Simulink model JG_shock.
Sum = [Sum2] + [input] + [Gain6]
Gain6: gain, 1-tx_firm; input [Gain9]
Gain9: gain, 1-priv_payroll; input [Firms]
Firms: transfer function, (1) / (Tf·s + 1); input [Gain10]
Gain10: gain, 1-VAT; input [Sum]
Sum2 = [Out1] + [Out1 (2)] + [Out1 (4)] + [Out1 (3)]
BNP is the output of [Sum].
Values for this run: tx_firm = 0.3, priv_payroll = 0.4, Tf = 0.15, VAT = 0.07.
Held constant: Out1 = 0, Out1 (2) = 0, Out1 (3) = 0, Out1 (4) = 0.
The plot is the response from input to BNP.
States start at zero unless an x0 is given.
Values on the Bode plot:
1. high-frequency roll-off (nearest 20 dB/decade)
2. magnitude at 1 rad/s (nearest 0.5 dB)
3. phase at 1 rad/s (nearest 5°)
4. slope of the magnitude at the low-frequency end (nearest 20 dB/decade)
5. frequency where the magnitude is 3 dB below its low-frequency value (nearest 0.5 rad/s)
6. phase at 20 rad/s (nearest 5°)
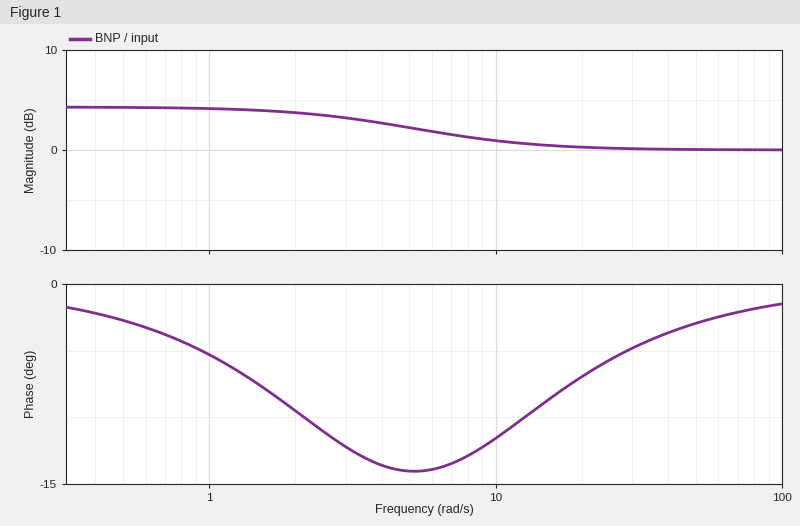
0 dB/decade
4.0 dB
-5°
0 dB/decade
8.0 rad/s
-5°
